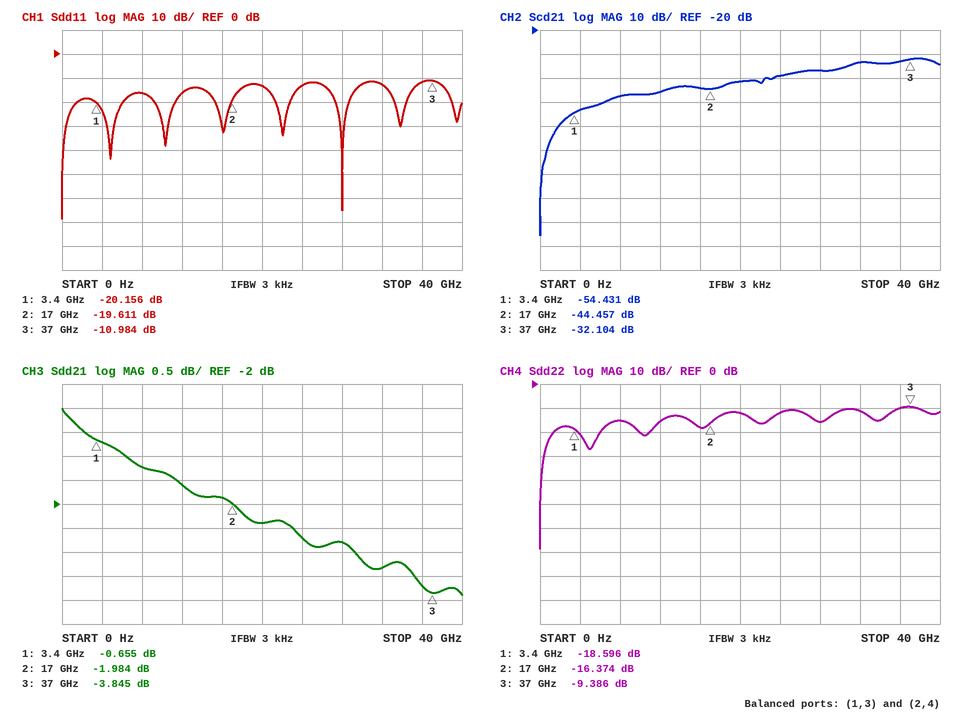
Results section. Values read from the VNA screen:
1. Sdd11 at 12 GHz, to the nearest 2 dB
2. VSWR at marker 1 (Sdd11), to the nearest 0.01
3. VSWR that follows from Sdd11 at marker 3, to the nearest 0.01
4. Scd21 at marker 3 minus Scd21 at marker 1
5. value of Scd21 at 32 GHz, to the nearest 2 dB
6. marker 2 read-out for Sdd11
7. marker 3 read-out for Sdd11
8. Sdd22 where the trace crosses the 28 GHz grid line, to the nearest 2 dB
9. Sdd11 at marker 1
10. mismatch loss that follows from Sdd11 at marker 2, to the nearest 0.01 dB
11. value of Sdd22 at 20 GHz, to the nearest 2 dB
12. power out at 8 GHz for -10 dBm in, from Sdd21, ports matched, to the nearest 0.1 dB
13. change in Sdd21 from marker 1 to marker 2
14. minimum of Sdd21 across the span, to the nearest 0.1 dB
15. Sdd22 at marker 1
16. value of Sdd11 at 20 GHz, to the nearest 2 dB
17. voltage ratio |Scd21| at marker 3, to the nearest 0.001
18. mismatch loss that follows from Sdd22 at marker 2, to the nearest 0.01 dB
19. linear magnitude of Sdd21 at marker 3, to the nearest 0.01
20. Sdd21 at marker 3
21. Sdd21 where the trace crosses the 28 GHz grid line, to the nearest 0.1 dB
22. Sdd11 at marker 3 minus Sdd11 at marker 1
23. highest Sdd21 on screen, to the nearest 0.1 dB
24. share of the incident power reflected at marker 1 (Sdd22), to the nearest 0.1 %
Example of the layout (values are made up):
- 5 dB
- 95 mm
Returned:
- -16 dB
- 1.22
- 1.79
- 22.327 dB
- -34 dB
- -19.611 dB
- -10.984 dB
- -16 dB
- -20.156 dB
- 0.05 dB
- -12 dB
- -11.2 dBm
- -1.329 dB
- -3.9 dB
- -18.596 dB
- -14 dB
- 0.025
- 0.10 dB
- 0.64
- -3.845 dB
- -2.8 dB
- 9.172 dB
- 0.0 dB
- 1.4 %
